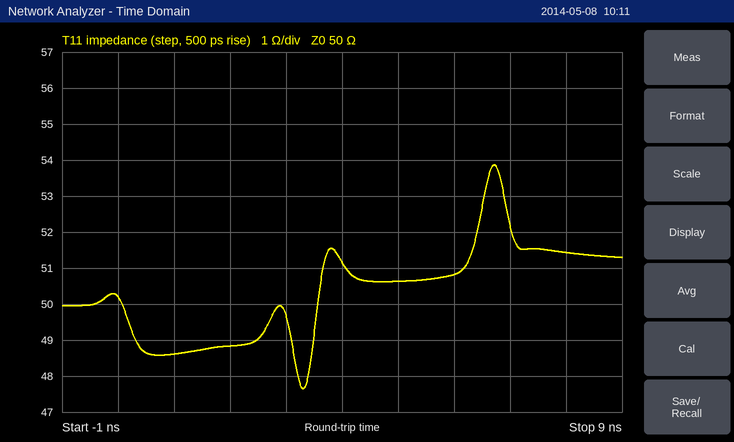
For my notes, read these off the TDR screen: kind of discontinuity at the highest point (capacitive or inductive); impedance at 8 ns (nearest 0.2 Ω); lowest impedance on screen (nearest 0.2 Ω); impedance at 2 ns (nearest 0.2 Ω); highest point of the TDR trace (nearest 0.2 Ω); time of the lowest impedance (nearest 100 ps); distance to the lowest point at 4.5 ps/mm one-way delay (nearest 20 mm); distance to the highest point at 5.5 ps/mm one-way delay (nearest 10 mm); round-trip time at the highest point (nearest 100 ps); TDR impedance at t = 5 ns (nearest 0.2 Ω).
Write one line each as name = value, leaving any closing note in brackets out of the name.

kind of discontinuity at the highest point = inductive
impedance at 8 ns = 51.4 Ω
lowest impedance on screen = 47.6 Ω
impedance at 2 ns = 48.8 Ω
highest point of the TDR trace = 53.8 Ω
time of the lowest impedance = 3.3 ns
distance to the lowest point at 4.5 ps/mm one-way delay = 360 mm
distance to the highest point at 5.5 ps/mm one-way delay = 610 mm
round-trip time at the highest point = 6.7 ns
TDR impedance at t = 5 ns = 50.6 Ω
